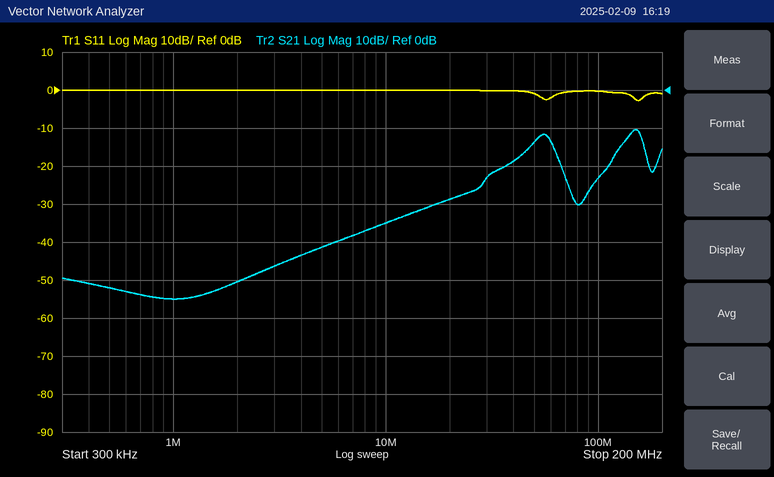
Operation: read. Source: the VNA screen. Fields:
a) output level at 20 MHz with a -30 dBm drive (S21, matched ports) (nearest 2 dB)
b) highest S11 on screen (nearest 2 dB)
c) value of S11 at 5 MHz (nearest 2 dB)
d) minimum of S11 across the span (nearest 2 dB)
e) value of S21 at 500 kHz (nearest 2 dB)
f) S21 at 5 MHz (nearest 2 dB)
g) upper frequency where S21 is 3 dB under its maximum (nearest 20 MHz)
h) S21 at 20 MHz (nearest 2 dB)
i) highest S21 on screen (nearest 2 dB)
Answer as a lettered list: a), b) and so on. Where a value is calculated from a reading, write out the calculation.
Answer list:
a) -30 dBm + (-28 dB) = -58 dBm
b) 0 dB
c) 0 dB
d) -2 dB
e) -52 dB
f) -42 dB
g) 160 MHz
h) -28 dB
i) -10 dB
